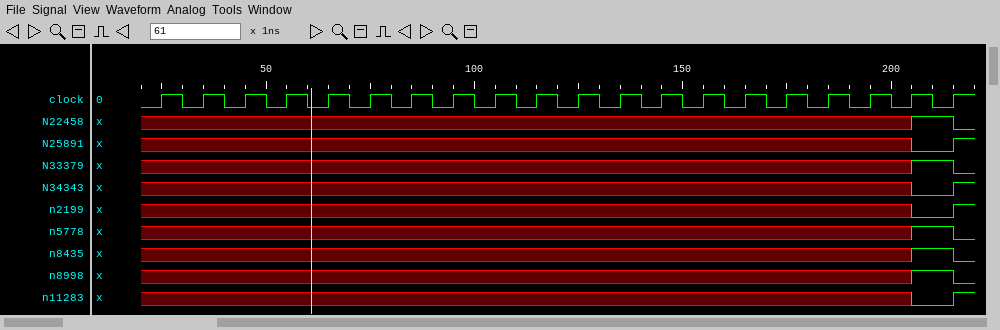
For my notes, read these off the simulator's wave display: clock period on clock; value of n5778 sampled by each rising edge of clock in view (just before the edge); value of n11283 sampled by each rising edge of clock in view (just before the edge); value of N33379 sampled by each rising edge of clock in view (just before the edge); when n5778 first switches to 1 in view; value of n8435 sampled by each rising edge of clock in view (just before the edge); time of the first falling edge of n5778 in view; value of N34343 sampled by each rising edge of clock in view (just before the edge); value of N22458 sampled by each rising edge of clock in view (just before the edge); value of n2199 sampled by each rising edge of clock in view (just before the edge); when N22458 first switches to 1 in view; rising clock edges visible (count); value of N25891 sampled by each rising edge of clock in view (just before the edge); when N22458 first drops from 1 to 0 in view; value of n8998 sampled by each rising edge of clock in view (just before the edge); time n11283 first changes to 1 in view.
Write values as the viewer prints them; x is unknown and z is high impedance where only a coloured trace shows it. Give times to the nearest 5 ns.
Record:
10 ns
x x x x x x x x x x x x x x x x x x x 1
x x x x x x x x x x x x x x x x x x x 0
x x x x x x x x x x x x x x x x x x x 1
205 ns
x x x x x x x x x x x x x x x x x x x 1
215 ns
x x x x x x x x x x x x x x x x x x x 0
x x x x x x x x x x x x x x x x x x x 1
x x x x x x x x x x x x x x x x x x x 0
205 ns
20
x x x x x x x x x x x x x x x x x x x 0
215 ns
x x x x x x x x x x x x x x x x x x x 1
215 ns
